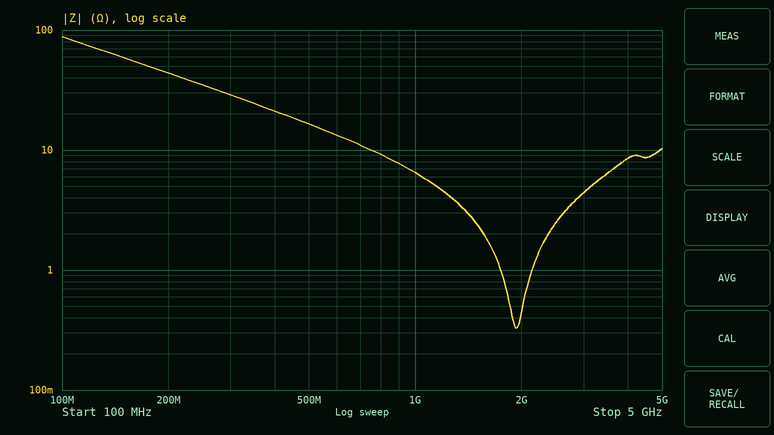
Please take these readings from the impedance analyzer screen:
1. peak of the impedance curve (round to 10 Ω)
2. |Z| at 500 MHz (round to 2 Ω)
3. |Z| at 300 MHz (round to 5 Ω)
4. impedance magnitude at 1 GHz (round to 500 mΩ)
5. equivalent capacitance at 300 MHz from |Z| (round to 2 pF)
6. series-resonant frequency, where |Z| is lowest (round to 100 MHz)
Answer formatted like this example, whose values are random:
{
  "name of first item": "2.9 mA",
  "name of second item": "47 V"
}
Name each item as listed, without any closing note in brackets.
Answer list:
{
  "peak of the impedance curve": "90 Ω",
  "|Z| at 500 MHz": "16 Ω",
  "|Z| at 300 MHz": "30 Ω",
  "impedance magnitude at 1 GHz": "6.5 Ω",
  "equivalent capacitance at 300 MHz from |Z|": "18 pF",
  "series-resonant frequency, where |Z| is lowest": "1.9 GHz"
}
